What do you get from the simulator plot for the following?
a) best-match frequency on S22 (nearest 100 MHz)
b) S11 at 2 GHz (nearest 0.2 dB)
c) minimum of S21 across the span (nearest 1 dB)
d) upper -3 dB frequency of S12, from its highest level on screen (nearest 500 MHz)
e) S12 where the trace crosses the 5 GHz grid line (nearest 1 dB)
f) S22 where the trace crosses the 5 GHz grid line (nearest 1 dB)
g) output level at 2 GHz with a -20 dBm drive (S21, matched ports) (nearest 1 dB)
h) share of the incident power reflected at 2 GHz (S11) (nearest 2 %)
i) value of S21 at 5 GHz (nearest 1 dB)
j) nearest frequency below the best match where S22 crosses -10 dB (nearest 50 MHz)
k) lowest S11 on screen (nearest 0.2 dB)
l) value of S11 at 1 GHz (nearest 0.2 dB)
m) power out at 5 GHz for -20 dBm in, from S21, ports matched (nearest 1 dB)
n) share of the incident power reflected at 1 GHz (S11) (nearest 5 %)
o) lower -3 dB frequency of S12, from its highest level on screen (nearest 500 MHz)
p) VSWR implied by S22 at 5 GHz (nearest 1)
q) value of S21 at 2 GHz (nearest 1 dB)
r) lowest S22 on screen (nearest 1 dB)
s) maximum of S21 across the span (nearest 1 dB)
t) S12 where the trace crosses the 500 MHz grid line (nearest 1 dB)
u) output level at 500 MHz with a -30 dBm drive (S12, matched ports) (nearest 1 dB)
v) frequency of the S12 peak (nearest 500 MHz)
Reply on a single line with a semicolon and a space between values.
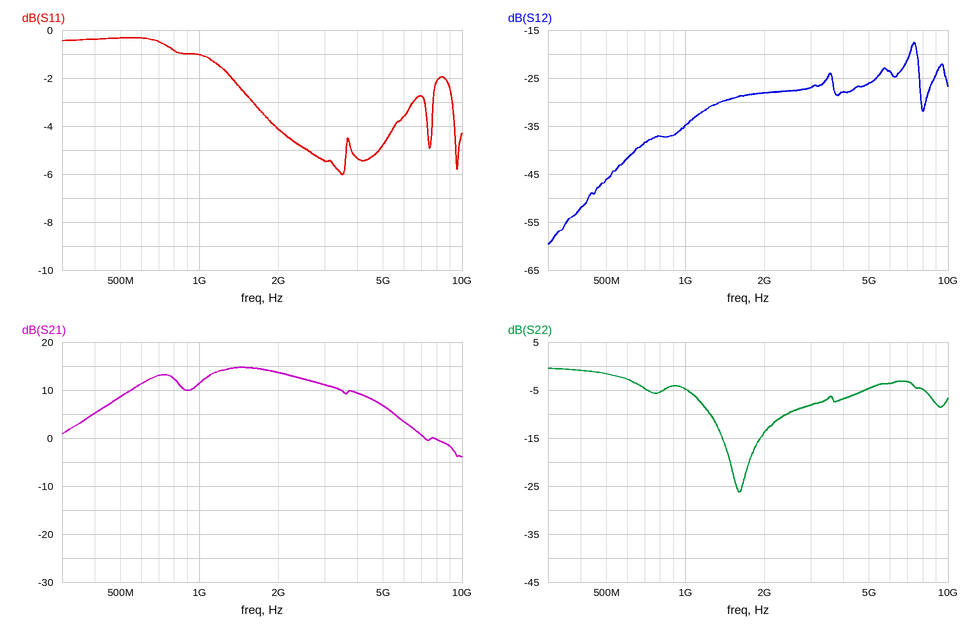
1.6 GHz; -4.2 dB; -4 dB; 7.5 GHz; -26 dB; -5 dB; -6 dBm; 38 %; 7 dB; 1.25 GHz; -6.0 dB; -1.0 dB; -13 dBm; 80 %; 7.0 GHz; 4; 14 dB; -26 dB; 15 dB; -46 dB; -76 dBm; 7.5 GHz
